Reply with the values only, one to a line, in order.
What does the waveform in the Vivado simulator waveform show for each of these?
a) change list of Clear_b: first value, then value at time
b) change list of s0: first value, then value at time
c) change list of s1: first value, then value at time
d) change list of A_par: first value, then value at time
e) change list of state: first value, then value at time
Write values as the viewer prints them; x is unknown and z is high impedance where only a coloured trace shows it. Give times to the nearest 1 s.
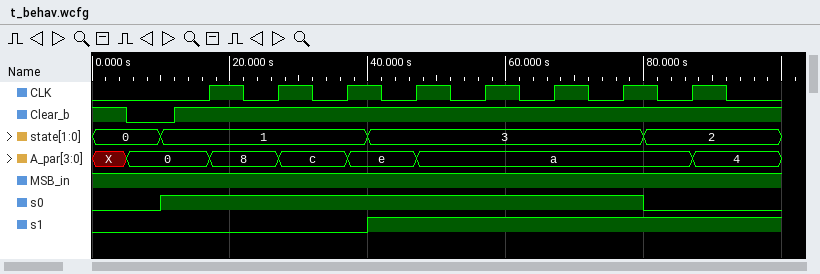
1, 0 at 5 s, 1 at 12 s
0, 1 at 10 s, 0 at 80 s
0, 1 at 40 s
X, 0 at 5 s, 8 at 17 s, c at 27 s, e at 37 s, a at 47 s, 4 at 87 s
0, 1 at 10 s, 3 at 40 s, 2 at 80 s
